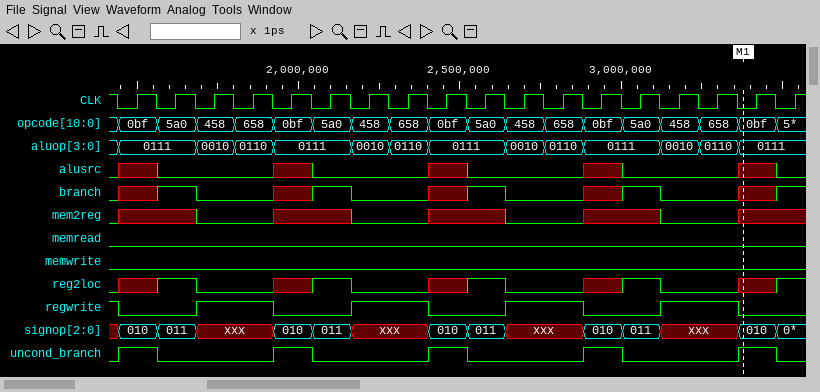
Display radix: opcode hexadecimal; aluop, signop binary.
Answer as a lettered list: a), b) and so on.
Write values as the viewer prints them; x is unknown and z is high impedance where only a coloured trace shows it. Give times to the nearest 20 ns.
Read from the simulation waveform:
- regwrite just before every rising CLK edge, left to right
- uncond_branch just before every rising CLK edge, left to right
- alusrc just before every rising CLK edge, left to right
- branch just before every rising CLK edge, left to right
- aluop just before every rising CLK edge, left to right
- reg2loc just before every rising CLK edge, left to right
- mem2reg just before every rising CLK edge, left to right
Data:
a) 0 0 1 1 0 0 1 1 0 0 1 1 0 0 1 1 0 0
b) 1 0 0 0 1 0 0 0 1 0 0 0 1 0 0 0 1 0
c) x 0 0 0 x 0 0 0 x 0 0 0 x 0 0 0 x 0
d) x 1 0 0 x 1 0 0 x 1 0 0 x 1 0 0 x 1
e) 0111, 0111, 0010, 0110, 0111, 0111, 0010, 0110, 0111, 0111, 0010, 0110, 0111, 0111, 0010, 0110, 0111, 0111
f) x 1 0 0 x 1 0 0 x 1 0 0 x 1 0 0 x 1
g) x x 0 0 x x 0 0 x x 0 0 x x 0 0 x x
